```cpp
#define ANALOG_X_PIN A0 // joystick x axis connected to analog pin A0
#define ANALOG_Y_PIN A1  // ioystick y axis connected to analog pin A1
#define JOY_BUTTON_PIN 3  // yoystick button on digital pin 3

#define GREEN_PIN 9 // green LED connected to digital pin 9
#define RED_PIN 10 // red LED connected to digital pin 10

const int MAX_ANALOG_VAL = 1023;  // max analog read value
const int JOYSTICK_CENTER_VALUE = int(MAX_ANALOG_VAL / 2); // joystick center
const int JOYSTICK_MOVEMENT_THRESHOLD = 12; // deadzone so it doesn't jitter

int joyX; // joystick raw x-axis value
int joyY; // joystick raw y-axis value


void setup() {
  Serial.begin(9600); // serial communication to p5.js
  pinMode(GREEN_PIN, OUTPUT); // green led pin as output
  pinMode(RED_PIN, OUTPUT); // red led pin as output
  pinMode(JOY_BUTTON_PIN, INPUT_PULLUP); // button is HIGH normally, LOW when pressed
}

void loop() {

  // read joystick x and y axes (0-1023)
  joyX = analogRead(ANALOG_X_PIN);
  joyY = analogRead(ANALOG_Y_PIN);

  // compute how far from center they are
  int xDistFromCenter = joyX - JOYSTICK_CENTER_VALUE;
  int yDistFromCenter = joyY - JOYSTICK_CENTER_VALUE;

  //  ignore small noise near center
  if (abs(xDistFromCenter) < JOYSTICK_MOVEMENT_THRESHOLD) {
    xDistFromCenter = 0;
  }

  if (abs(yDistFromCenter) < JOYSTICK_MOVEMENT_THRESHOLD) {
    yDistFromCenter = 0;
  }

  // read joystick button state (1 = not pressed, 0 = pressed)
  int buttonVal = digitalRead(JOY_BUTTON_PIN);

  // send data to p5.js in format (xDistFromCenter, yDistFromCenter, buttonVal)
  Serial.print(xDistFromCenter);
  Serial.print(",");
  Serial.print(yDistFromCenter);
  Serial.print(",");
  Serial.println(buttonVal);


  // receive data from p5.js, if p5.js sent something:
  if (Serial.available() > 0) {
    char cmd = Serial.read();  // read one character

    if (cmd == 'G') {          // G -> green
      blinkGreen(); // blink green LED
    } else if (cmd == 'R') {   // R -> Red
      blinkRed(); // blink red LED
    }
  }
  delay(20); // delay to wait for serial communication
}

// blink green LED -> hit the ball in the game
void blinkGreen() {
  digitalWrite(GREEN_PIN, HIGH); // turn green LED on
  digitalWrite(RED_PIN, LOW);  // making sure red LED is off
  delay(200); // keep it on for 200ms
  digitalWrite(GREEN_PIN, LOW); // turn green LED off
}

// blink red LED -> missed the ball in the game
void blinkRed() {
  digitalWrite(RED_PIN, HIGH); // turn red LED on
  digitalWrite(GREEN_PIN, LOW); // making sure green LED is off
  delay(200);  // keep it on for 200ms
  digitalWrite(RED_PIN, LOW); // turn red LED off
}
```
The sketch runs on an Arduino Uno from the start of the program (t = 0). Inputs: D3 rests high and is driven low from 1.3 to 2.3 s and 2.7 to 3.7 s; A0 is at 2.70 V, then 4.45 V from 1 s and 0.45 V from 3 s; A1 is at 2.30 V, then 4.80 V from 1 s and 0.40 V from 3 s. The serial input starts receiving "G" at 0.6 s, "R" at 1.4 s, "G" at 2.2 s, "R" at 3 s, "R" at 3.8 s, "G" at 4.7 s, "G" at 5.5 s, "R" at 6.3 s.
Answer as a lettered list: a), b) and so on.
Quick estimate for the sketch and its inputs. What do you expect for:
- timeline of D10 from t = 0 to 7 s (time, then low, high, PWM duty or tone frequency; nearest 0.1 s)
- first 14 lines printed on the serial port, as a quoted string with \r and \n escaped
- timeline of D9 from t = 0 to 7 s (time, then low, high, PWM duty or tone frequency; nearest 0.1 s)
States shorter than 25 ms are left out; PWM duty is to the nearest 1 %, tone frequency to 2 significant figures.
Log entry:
a) 0 s low; 1.4 s high; 1.6 s low; 3 s high; 3.2 s low; 3.8 s high; 4 s low; 6.3 s high; 6.5 s low
b) "41,-40,1\r\n41,-40,1\r\n41,-40,1\r\n41,-40,1\r\n41,-40,1\r\n41,-40,1\r\n41,-40,1\r\n41,-40,1\r\n41,-40,1\r\n41,-40,1\r\n41,-40,1\r\n41,-40,1\r\n41,-40,1\r\n41,-40,1\r\n"
c) 0 s low; 0.6 s high; 0.8 s low; 2.2 s high; 2.4 s low; 4.7 s high; 4.9 s low; 5.5 s high; 5.7 s low
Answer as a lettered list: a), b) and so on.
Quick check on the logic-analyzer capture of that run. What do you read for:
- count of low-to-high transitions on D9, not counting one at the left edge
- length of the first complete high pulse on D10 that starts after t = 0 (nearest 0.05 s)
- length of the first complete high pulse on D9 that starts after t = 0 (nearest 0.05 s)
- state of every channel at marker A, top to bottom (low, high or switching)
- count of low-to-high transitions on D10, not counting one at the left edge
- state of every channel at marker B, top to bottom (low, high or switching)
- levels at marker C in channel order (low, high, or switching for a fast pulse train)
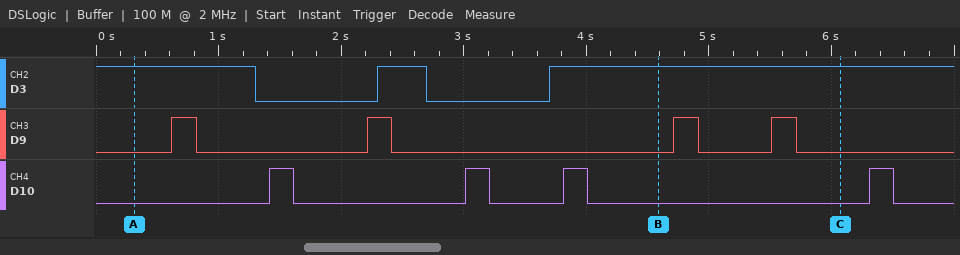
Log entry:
a) 4
b) 0.20 s
c) 0.20 s
d) D3 high, D9 low, D10 low
e) 4
f) D3 high, D9 low, D10 low
g) D3 high, D9 low, D10 low
